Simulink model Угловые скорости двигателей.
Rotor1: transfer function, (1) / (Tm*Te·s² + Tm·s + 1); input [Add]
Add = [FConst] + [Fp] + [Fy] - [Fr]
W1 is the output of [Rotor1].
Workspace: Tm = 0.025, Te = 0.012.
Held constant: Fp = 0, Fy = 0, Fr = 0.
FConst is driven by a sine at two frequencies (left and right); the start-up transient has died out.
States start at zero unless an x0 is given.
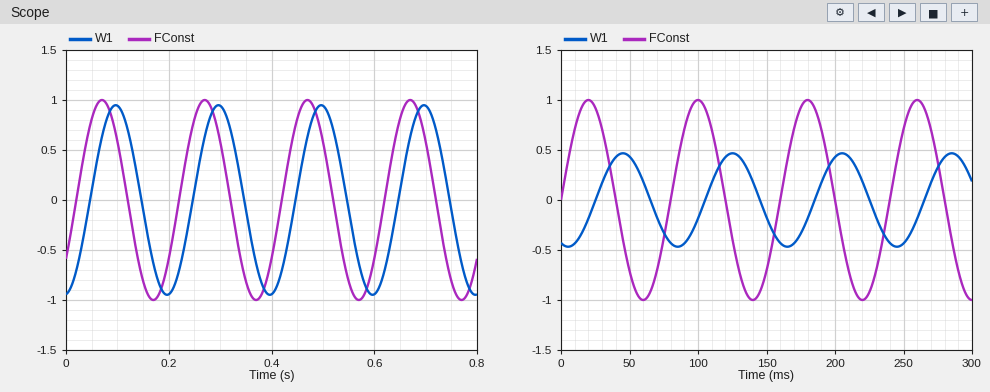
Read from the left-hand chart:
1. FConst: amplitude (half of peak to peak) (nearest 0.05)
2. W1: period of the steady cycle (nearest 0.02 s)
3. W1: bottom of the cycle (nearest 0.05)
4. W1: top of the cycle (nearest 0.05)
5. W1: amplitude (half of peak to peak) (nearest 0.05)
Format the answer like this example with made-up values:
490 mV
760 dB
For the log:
1.00
0.20 s
-0.95
0.95
0.95
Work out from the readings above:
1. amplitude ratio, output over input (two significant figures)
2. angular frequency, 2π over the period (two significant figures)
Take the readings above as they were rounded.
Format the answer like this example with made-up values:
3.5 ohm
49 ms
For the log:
0.95
31 rad/s
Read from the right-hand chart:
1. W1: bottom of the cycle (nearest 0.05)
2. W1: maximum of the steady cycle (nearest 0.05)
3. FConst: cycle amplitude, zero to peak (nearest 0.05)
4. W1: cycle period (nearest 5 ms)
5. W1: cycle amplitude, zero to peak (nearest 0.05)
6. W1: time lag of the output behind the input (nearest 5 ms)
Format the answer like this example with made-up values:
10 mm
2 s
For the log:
-0.45
0.45
1.00
80 ms
0.45
25 ms
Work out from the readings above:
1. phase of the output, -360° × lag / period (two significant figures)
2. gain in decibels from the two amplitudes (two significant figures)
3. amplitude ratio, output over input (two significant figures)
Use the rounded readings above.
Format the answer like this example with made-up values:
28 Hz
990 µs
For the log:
-110°
-6.9 dB
0.45
